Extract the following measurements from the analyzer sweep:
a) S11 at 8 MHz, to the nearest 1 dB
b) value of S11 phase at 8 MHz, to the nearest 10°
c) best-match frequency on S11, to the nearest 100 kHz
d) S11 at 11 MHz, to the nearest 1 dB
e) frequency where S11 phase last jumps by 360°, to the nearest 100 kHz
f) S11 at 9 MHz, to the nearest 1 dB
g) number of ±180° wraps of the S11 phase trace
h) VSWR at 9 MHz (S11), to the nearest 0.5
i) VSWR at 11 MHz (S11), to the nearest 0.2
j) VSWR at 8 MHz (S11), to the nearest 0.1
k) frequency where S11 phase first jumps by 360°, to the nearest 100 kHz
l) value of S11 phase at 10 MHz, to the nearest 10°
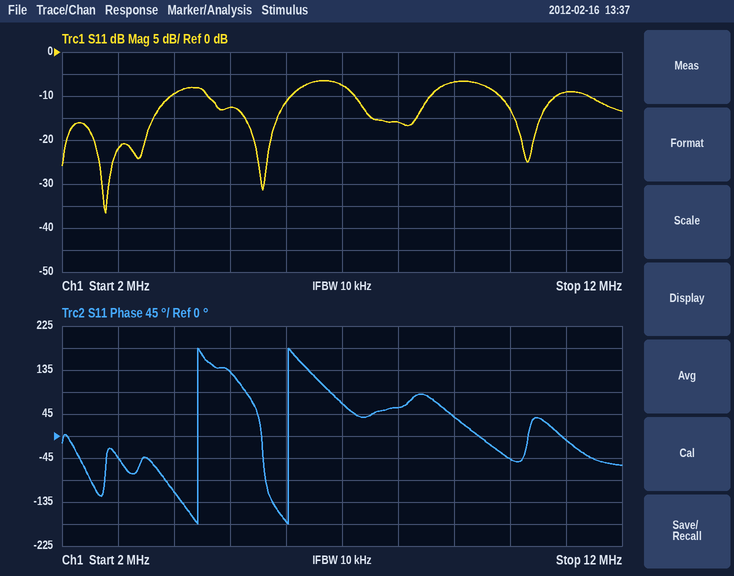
-16 dB
60°
2.8 MHz
-9 dB
6.0 MHz
-7 dB
2
2.5
2.0
1.4
4.4 MHz
-50°
